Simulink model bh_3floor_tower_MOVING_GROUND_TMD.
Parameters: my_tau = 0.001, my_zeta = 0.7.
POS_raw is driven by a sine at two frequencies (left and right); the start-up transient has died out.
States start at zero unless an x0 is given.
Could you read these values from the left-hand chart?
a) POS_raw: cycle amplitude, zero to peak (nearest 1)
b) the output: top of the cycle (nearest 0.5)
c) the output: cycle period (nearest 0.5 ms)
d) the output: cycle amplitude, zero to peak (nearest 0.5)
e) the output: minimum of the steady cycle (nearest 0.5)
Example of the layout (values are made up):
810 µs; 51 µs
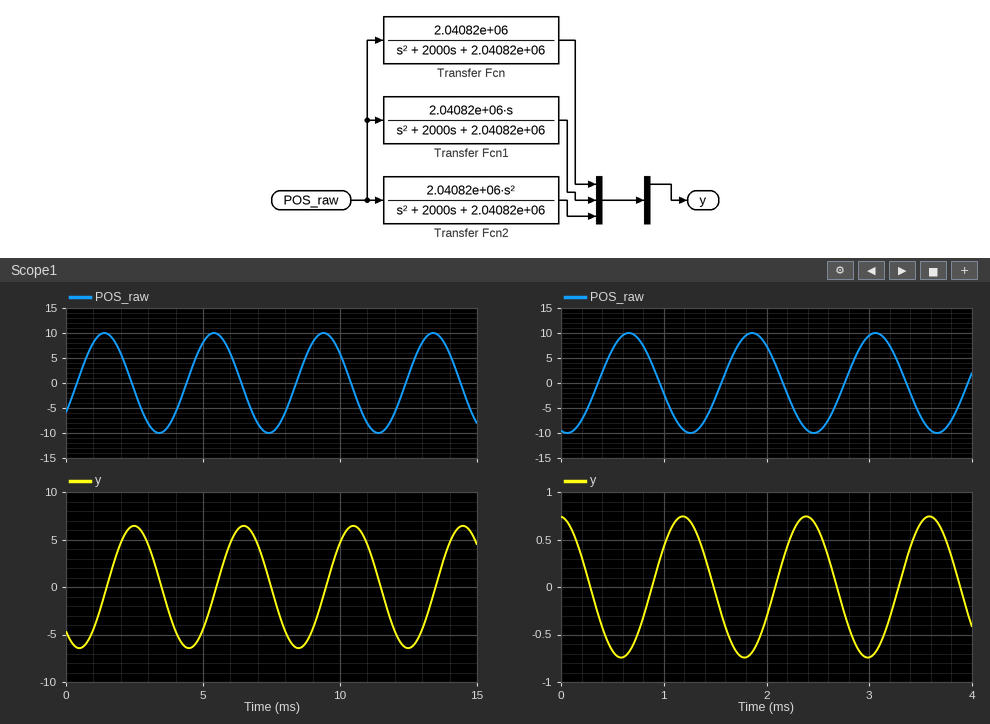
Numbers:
10; 6.5; 4.0 ms; 6.5; -6.5
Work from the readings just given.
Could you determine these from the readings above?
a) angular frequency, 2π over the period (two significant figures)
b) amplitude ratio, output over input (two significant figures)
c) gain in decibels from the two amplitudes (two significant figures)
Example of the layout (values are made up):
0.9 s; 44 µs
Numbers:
1.6 rad/ms; 0.65; -3.7 dB
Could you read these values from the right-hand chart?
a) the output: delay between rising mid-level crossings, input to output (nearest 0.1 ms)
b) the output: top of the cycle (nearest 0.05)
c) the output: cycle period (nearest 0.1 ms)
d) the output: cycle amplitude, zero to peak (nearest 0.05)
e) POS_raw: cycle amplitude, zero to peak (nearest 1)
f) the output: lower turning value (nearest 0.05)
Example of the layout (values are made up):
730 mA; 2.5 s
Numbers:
0.5 ms; 0.75; 1.2 ms; 0.75; 10; -0.75
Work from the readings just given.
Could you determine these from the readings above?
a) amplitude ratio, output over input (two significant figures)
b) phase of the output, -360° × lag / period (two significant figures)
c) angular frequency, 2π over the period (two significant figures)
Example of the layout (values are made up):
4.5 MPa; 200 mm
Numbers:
0.075; -150°; 5.2 rad/ms
